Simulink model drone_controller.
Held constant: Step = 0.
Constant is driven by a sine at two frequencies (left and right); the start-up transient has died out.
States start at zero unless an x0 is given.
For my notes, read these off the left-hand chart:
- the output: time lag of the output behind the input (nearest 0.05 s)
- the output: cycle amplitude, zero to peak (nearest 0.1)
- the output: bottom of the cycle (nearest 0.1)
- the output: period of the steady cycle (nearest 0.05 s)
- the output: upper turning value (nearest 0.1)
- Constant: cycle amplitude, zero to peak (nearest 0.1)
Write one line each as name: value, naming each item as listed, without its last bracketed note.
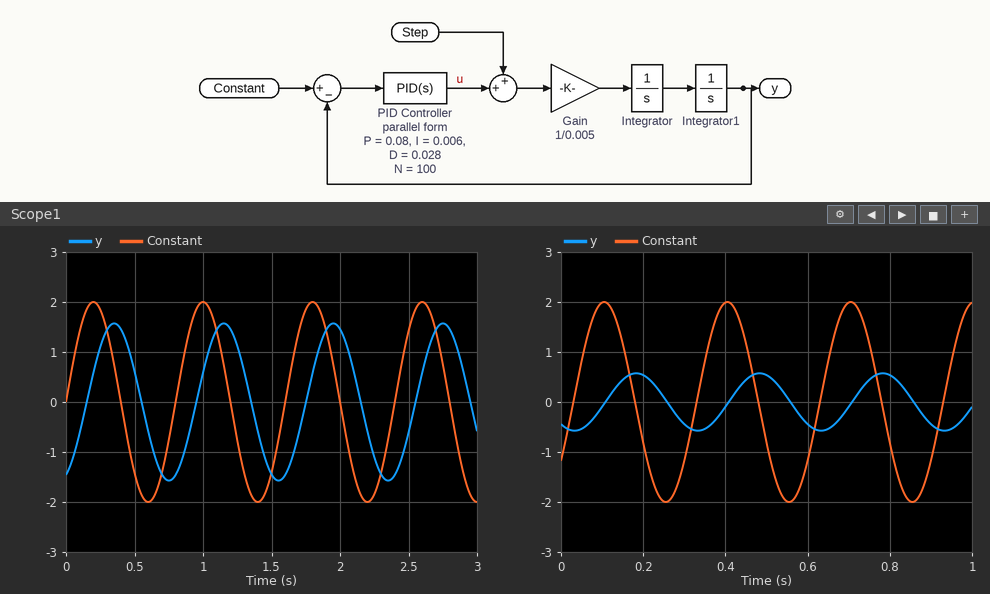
the output: time lag of the output behind the input: 0.15 s
the output: cycle amplitude, zero to peak: 1.6
the output: bottom of the cycle: -1.6
the output: period of the steady cycle: 0.80 s
the output: upper turning value: 1.6
Constant: cycle amplitude, zero to peak: 2.0
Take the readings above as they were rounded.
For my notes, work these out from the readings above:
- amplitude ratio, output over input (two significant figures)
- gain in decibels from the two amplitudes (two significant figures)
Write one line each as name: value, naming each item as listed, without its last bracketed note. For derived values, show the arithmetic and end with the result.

amplitude ratio, output over input: 1.6 / 2 = 0.80
gain in decibels from the two amplitudes: 20 log10(1.6 / 2) = -1.9 dB
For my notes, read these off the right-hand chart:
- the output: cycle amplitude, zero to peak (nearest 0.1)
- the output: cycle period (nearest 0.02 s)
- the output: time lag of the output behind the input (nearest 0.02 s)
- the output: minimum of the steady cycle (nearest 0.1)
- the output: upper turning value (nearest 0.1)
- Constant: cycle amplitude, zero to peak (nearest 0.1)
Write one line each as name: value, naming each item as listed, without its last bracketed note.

the output: cycle amplitude, zero to peak: 0.6
the output: cycle period: 0.30 s
the output: time lag of the output behind the input: 0.08 s
the output: minimum of the steady cycle: -0.6
the output: upper turning value: 0.6
Constant: cycle amplitude, zero to peak: 2.0
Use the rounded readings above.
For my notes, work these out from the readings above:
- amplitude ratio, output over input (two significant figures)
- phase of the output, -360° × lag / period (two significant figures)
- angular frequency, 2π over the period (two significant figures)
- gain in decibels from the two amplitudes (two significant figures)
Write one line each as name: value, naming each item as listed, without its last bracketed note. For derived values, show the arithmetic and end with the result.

amplitude ratio, output over input: 0.6 / 2 = 0.30
phase of the output, -360° × lag / period: -360 × 0.08 / 0.3 = -96°
angular frequency, 2π over the period: 2π / 0.3 = 21 rad/s
gain in decibels from the two amplitudes: 20 log10(0.6 / 2) = -10 dB
